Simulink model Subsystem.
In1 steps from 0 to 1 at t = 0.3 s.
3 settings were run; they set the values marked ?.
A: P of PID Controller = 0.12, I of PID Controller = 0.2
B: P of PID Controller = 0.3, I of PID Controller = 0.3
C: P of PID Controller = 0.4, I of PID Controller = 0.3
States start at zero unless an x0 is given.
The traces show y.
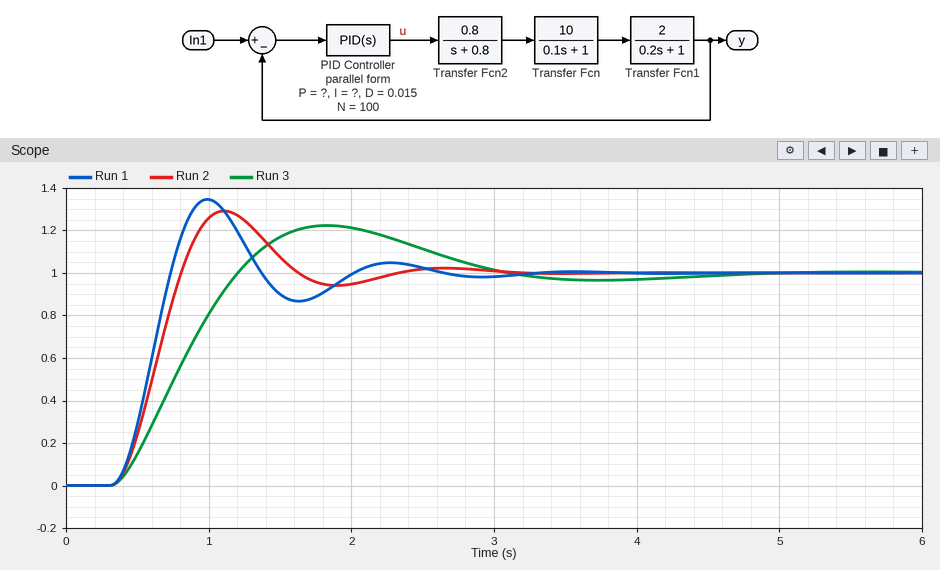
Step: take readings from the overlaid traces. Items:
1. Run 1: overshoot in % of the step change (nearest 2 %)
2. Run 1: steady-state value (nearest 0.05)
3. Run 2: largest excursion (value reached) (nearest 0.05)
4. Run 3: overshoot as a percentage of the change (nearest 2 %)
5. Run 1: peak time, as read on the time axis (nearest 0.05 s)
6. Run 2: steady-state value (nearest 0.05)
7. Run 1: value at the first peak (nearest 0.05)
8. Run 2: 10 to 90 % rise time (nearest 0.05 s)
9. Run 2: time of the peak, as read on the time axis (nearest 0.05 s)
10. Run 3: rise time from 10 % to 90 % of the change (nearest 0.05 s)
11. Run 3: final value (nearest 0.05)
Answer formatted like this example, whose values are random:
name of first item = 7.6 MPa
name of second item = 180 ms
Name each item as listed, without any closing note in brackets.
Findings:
Run 1: overshoot in % of the step change = 34 %
Run 1: steady-state value = 1.00
Run 2: largest excursion (value reached) = 1.30
Run 3: overshoot as a percentage of the change = 22 %
Run 1: peak time, as read on the time axis = 1.00 s
Run 2: steady-state value = 1.00
Run 1: value at the first peak = 1.35
Run 2: 10 to 90 % rise time = 0.35 s
Run 2: time of the peak, as read on the time axis = 1.10 s
Run 3: rise time from 10 % to 90 % of the change = 0.65 s
Run 3: final value = 1.00
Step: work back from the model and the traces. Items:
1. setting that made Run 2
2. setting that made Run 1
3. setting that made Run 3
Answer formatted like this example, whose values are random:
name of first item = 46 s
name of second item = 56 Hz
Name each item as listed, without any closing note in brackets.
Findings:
setting that made Run 2 = B
setting that made Run 1 = C
setting that made Run 3 = A
